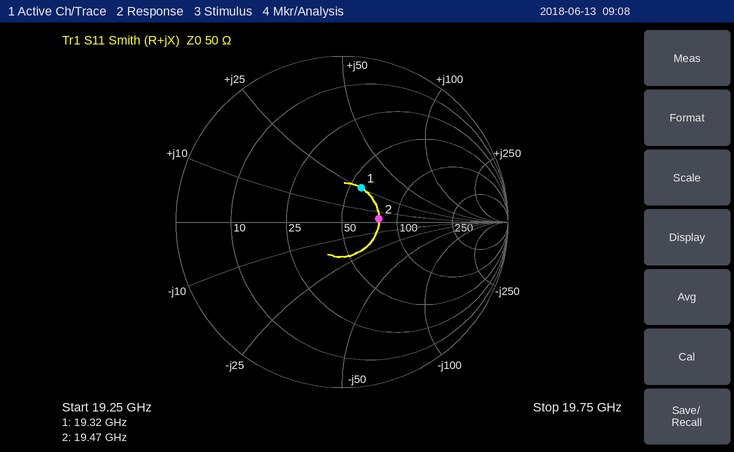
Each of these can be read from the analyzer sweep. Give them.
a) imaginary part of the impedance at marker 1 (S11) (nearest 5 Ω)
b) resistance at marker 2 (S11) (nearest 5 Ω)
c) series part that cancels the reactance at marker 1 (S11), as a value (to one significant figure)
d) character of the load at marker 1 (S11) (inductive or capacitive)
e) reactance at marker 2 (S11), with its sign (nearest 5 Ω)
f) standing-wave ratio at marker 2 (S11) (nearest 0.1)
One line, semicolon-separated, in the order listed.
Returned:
+25 Ω; 80 Ω; 300 fF; inductive; +5 Ω; 1.6
